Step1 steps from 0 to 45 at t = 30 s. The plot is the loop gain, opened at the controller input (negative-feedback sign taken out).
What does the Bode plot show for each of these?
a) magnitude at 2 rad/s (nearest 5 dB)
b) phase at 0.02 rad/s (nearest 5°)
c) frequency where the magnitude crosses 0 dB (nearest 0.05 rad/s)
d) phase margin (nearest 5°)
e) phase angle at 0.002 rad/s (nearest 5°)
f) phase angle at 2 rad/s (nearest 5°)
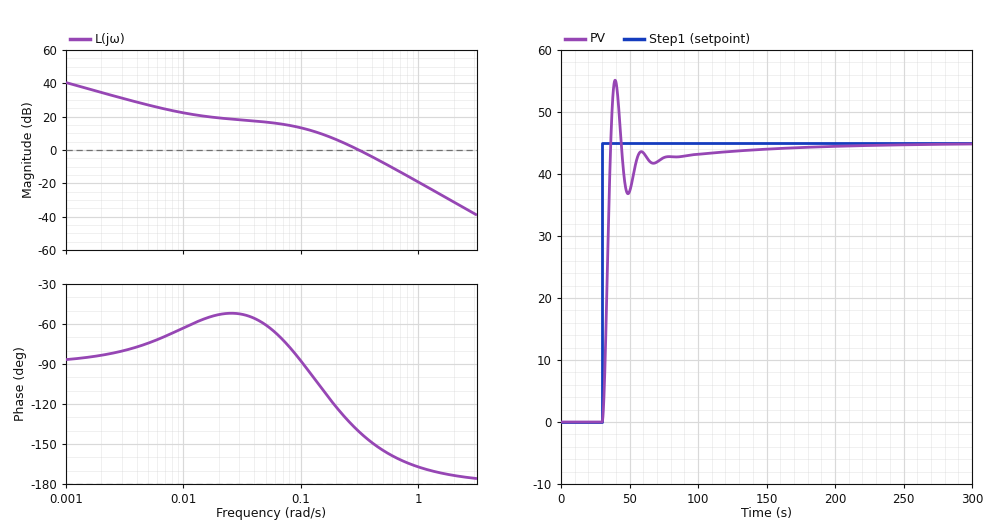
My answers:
-30 dB
-55°
0.30 rad/s
40°
-85°
-175°
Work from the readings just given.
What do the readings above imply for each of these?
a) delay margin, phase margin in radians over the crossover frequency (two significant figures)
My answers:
2.3 s
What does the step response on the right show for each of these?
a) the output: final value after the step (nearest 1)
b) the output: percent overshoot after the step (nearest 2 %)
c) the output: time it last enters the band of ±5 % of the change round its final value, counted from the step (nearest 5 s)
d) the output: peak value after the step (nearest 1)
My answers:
45
22 %
45 s
55
